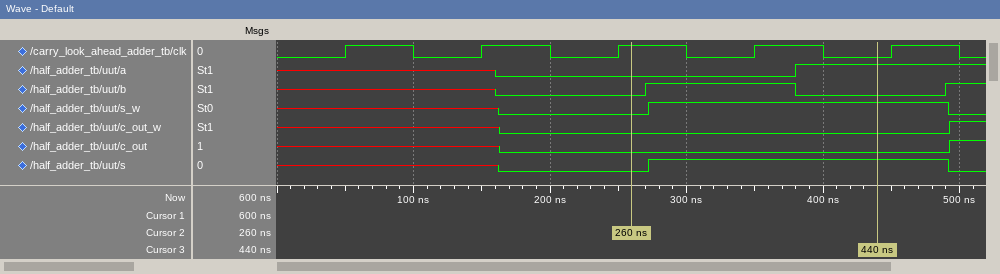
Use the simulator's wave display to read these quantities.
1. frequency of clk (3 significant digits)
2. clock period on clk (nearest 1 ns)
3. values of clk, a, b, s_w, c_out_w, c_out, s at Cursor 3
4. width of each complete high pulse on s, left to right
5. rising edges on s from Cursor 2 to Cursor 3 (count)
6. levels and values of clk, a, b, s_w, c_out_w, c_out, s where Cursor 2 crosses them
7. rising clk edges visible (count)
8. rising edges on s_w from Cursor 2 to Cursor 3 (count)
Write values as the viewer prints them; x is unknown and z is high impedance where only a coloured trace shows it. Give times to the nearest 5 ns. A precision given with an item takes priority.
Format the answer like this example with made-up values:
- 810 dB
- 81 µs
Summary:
- 10.0 MHz
- 100 ns
- clk=0, a=1, b=0, s_w=1, c_out_w=0, c_out=0, s=1
- 220 ns
- 1
- clk=1, a=0, b=0, s_w=0, c_out_w=0, c_out=0, s=0
- 5
- 1
